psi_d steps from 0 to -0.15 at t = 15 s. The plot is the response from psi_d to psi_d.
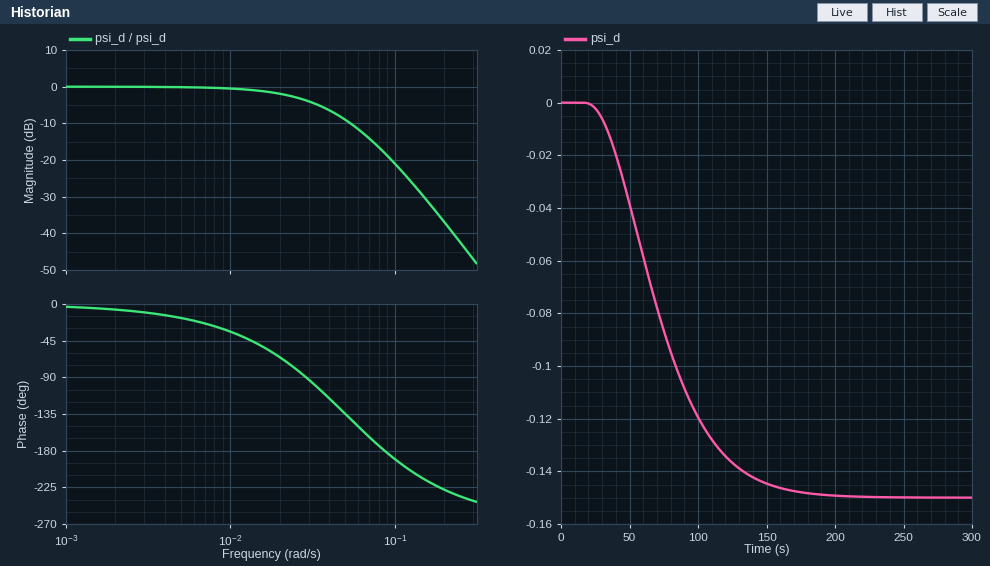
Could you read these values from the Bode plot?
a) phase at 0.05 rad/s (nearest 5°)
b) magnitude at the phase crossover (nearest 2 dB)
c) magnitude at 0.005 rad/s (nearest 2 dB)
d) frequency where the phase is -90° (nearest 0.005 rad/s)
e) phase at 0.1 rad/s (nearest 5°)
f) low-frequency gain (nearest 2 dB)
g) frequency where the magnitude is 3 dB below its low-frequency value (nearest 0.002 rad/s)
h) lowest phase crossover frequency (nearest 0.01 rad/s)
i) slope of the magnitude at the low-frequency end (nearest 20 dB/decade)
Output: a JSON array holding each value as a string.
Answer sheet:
["-135°", "-18 dB", "0 dB", "0.030 rad/s", "-190°", "0 dB", "0.026 rad/s", "0.09 rad/s", "0 dB/decade"]
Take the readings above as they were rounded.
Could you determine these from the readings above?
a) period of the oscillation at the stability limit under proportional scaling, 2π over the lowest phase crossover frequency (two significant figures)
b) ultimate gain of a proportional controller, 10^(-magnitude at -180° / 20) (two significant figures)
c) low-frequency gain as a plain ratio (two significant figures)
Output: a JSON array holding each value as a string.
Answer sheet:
["70 s", "7.9", "1.0"]
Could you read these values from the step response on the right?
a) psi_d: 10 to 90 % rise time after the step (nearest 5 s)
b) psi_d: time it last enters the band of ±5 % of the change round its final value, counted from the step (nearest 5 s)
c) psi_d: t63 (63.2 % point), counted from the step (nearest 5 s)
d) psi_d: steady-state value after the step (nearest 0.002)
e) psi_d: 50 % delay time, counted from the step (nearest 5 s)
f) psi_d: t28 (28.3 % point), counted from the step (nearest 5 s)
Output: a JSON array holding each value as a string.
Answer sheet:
["85 s", "125 s", "65 s", "-0.150", "55 s", "35 s"]
